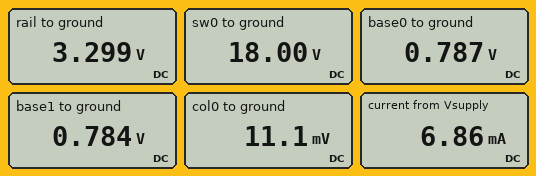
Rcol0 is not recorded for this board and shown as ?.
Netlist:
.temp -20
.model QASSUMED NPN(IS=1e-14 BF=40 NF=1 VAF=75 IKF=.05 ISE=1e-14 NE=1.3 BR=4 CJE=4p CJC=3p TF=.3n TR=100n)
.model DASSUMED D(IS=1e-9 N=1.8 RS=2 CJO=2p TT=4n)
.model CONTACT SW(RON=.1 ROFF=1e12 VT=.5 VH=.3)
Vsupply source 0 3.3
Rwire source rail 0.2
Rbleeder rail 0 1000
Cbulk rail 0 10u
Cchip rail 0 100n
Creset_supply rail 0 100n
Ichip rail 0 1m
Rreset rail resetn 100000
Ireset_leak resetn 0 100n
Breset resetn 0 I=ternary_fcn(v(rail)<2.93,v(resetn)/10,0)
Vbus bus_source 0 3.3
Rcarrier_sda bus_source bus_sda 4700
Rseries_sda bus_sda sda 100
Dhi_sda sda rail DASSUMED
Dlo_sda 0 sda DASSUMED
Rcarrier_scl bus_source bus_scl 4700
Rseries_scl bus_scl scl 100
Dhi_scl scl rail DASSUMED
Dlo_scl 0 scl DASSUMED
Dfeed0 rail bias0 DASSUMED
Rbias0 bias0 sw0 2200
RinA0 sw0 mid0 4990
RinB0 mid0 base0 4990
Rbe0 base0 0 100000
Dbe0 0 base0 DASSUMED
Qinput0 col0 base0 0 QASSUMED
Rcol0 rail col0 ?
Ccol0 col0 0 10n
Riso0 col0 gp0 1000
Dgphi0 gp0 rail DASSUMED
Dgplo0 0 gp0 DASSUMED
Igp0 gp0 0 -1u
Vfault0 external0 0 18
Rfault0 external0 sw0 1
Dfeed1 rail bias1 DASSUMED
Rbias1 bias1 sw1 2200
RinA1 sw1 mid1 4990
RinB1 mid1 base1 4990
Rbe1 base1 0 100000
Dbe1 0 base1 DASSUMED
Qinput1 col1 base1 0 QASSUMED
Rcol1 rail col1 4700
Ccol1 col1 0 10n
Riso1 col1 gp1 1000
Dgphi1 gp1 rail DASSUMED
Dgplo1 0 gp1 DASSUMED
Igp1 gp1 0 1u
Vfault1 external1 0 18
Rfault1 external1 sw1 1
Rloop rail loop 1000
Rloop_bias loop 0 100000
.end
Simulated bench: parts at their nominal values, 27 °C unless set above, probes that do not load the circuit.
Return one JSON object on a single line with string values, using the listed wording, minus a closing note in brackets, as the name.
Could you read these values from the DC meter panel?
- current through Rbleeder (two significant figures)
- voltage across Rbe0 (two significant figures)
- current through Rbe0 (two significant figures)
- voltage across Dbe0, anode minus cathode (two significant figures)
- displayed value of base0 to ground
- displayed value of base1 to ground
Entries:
{"current through Rbleeder": "3.3 mA", "voltage across Rbe0": "790 mV", "current through Rbe0": "7.9 µA", "voltage across Dbe0, anode minus cathode": "-790 mV", "displayed value of base0 to ground": "0.787 V", "displayed value of base1 to ground": "0.784 V"}
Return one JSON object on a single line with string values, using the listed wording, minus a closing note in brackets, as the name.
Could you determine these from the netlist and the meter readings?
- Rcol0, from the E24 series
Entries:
{"Rcol0, from the E24 series": "1.8 kΩ"}
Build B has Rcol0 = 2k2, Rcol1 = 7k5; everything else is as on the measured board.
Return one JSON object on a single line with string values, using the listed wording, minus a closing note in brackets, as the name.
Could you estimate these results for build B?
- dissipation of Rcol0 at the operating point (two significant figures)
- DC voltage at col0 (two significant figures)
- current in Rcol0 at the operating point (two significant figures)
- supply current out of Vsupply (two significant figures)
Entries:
{"dissipation of Rcol0 at the operating point": "4.9 mW", "DC voltage at col0": "10 mV", "current in Rcol0 at the operating point": "1.5 mA", "supply current out of Vsupply": "6.3 mA"}
